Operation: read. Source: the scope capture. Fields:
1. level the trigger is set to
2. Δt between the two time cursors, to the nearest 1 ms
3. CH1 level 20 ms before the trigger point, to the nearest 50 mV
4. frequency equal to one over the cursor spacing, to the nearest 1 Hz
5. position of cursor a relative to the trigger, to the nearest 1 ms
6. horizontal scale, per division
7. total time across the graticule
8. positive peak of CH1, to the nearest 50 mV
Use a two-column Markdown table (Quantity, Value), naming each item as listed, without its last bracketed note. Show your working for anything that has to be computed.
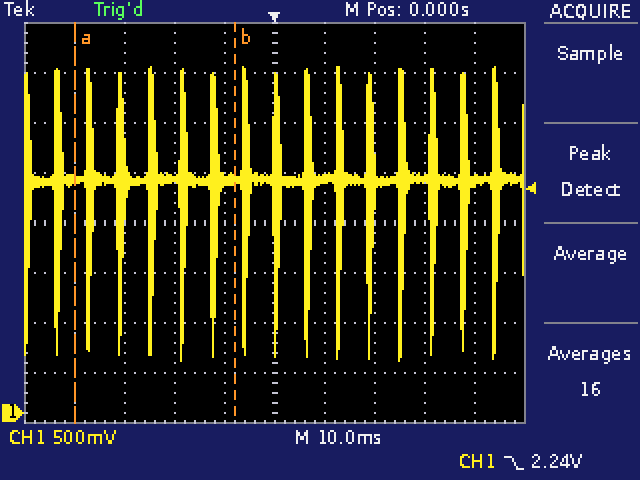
| Quantity | Value |
|---|---|
| level the trigger is set to | 2.24 V |
| Δt between the two time cursors, to the nearest 1 ms | 32 ms |
| CH1 level 20 ms before the trigger point, to the nearest 50 mV | 2.35 V |
| frequency equal to one over the cursor spacing, to the nearest 1 Hz | 1 / 32 ms ≈ 31 Hz |
| position of cursor a relative to the trigger, to the nearest 1 ms | -40 ms |
| horizontal scale, per division | 10 ms |
| total time across the graticule | 100 ms |
| positive peak of CH1, to the nearest 50 mV | 3.45 V |
